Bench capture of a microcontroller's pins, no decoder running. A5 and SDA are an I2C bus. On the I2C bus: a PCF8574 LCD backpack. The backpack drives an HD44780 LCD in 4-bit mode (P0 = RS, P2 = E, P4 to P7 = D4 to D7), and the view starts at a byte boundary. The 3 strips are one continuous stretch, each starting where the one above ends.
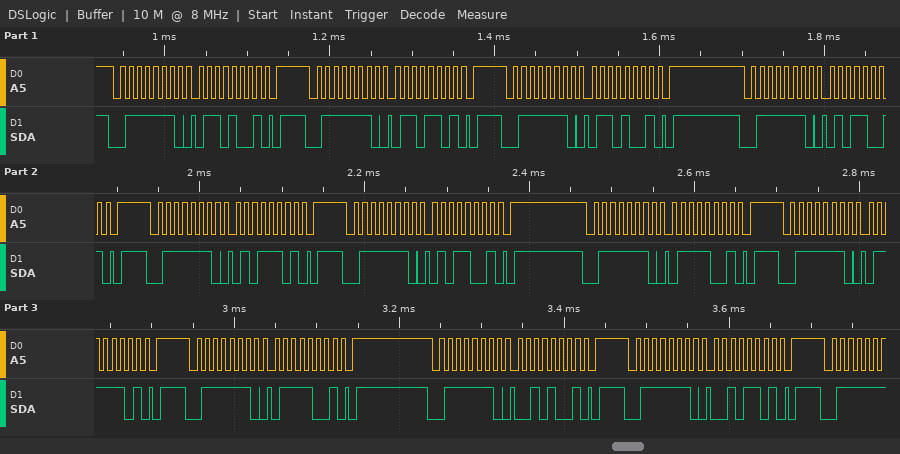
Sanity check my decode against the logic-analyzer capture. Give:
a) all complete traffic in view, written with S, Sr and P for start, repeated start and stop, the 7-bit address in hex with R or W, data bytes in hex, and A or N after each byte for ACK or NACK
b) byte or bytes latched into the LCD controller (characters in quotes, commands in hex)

S 3FW A 69 A P S 3FW A 6D A P S 3FW A 69 A P S 3FW A 59 A P S 3FW A 5D A P S 3FW A 59 A P S 3FW A 79 A P S 3FW A 7D A P S 3FW A 79 A P S 3FW A 29 A P S 3FW A 2D A P
'e'
